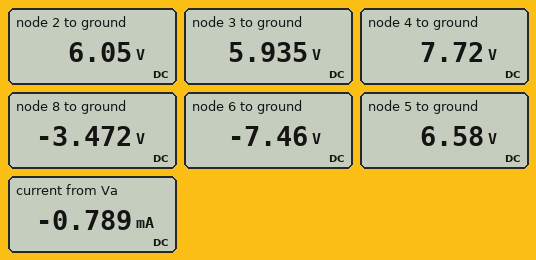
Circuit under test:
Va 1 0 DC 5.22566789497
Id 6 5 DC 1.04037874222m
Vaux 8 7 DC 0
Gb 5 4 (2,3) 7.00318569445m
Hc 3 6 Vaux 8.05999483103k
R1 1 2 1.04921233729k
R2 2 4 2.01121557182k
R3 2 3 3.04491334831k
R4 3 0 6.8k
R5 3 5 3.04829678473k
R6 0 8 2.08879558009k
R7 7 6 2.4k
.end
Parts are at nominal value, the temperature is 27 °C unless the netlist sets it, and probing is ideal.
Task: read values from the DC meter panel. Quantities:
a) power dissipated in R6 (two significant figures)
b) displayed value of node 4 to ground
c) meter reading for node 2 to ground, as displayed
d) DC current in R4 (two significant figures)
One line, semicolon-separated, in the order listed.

5.8 mW; 7.72 V; 6.05 V; 870 µA
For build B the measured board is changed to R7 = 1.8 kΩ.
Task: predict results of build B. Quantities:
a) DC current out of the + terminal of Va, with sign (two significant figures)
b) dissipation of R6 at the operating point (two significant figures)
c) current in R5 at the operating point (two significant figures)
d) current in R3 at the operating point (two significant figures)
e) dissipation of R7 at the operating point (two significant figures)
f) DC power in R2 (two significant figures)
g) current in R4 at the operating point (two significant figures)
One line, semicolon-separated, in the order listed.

-530 µA; 3.9 mW; 490 µA; 26 µA; 3.4 mW; 620 µW; 840 µA
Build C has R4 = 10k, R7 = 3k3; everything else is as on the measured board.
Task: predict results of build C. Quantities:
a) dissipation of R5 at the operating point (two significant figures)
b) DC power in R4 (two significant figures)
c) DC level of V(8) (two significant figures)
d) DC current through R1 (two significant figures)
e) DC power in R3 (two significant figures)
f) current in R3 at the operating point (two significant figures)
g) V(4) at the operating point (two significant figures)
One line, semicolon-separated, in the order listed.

2.8 mW; 4.8 mW; -5.4 V; 1.9 mA; 27 µW; 94 µA; 11 V
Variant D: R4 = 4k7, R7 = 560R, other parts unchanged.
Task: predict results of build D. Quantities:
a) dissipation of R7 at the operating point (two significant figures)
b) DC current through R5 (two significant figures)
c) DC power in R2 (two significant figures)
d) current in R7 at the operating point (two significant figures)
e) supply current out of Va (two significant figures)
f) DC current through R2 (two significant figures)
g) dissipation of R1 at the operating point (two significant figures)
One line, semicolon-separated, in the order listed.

500 µW; 1.2 mA; 45 µW; 940 µA; 140 µA; 150 µA; 21 µW
